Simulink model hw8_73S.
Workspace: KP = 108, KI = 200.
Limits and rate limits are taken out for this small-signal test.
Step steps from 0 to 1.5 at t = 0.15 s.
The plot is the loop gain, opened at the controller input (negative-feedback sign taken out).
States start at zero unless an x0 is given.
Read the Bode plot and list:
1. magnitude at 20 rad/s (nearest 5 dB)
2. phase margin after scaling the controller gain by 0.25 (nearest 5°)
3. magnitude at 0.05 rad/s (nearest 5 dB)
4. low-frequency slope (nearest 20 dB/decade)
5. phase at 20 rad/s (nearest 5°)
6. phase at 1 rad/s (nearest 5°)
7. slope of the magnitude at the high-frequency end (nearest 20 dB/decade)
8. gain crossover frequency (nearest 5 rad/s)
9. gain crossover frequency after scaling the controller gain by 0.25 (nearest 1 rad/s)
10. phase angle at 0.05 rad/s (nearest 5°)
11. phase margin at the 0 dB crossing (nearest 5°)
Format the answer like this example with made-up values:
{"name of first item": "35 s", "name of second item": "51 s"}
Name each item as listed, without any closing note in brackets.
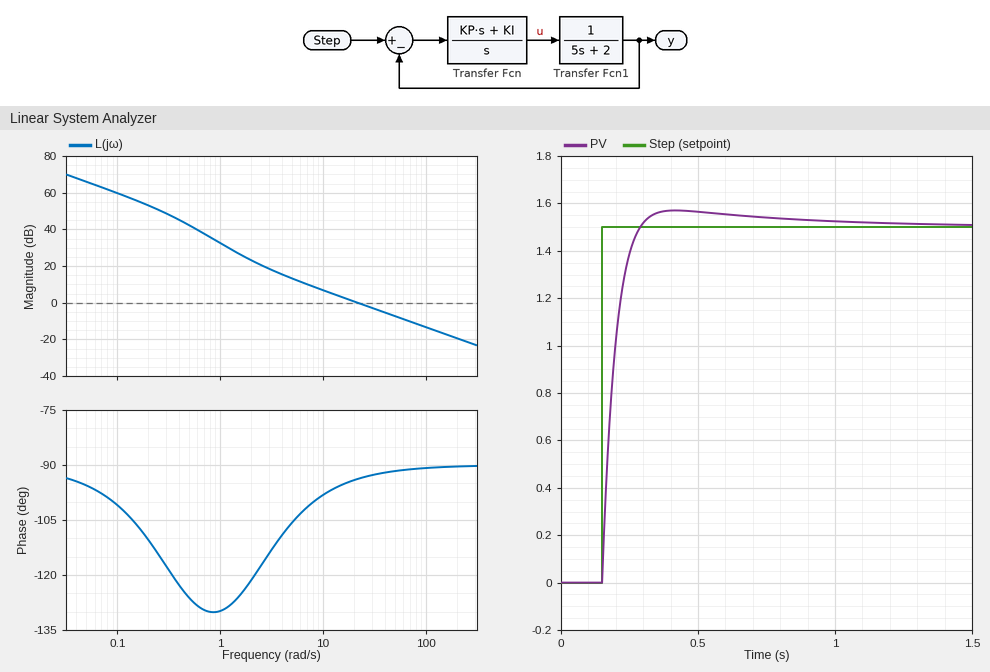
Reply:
{"magnitude at 20 rad/s": "0 dB", "phase margin after scaling the controller gain by 0.25": "75°", "magnitude at 0.05 rad/s": "65 dB", "low-frequency slope": "-20 dB/decade", "phase at 20 rad/s": "-95°", "phase at 1 rad/s": "-130°", "slope of the magnitude at the high-frequency end": "-20 dB/decade", "gain crossover frequency": "20 rad/s", "gain crossover frequency after scaling the controller gain by 0.25": "6 rad/s", "phase angle at 0.05 rad/s": "-95°", "phase margin at the 0 dB crossing": "85°"}
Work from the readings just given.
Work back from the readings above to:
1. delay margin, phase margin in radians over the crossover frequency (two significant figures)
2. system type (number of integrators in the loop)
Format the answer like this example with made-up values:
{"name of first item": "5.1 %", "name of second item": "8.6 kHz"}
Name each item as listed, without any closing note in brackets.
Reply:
{"delay margin, phase margin in radians over the crossover frequency": "0.074 s", "system type": "1"}
